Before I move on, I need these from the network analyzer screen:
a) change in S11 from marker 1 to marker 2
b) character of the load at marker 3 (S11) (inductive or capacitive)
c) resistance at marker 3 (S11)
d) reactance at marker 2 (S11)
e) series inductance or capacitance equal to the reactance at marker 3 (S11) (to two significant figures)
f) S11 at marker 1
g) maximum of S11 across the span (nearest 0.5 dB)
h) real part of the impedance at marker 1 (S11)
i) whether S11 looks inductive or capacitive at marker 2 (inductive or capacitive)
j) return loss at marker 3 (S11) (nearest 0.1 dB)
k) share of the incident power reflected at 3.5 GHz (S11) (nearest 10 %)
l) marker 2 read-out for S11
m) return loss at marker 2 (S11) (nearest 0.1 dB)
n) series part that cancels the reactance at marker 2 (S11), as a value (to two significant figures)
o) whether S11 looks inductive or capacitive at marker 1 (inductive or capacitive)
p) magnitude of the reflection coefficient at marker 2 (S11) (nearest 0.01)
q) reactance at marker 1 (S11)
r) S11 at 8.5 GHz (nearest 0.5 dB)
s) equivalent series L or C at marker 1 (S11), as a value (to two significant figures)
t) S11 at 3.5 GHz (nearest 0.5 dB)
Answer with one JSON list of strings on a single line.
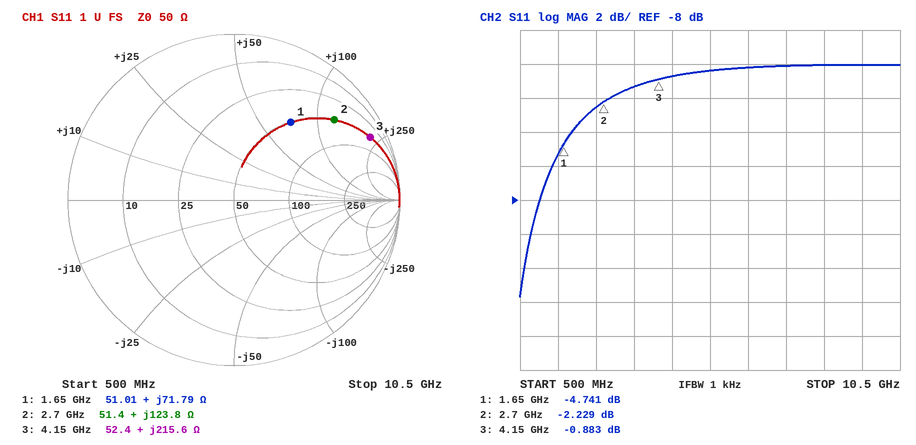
["2.512 dB", "inductive", "52.4 Ω", "+123.8 Ω", "8.3 nH", "-4.741 dB", "0.0 dB", "51.01 Ω", "inductive", "0.9 dB", "70 %", "-2.229 dB", "2.2 dB", "480 fF", "inductive", "0.77", "+71.79 Ω", "0.0 dB", "6.9 nH", "-1.5 dB"]
